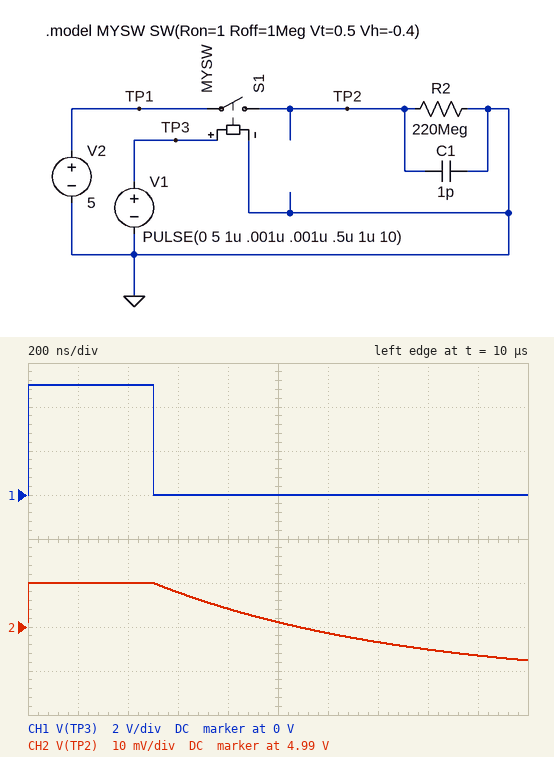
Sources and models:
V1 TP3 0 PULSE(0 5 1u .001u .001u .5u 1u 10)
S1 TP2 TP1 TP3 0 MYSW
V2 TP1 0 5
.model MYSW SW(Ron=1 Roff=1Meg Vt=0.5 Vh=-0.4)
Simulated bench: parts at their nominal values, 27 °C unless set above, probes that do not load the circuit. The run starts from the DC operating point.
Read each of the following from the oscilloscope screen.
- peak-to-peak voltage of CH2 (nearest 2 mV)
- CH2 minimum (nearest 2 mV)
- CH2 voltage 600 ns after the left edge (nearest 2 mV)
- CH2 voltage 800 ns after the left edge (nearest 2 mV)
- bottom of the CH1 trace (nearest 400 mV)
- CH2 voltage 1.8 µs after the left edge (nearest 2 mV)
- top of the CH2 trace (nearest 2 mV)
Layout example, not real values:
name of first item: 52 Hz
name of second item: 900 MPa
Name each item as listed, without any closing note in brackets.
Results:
peak-to-peak voltage of CH2: 18 mV
CH2 minimum: 4.982 V
CH2 voltage 600 ns after the left edge: 4.998 V
CH2 voltage 800 ns after the left edge: 4.994 V
bottom of the CH1 trace: 0 V
CH2 voltage 1.8 µs after the left edge: 4.984 V
top of the CH2 trace: 5.000 V
